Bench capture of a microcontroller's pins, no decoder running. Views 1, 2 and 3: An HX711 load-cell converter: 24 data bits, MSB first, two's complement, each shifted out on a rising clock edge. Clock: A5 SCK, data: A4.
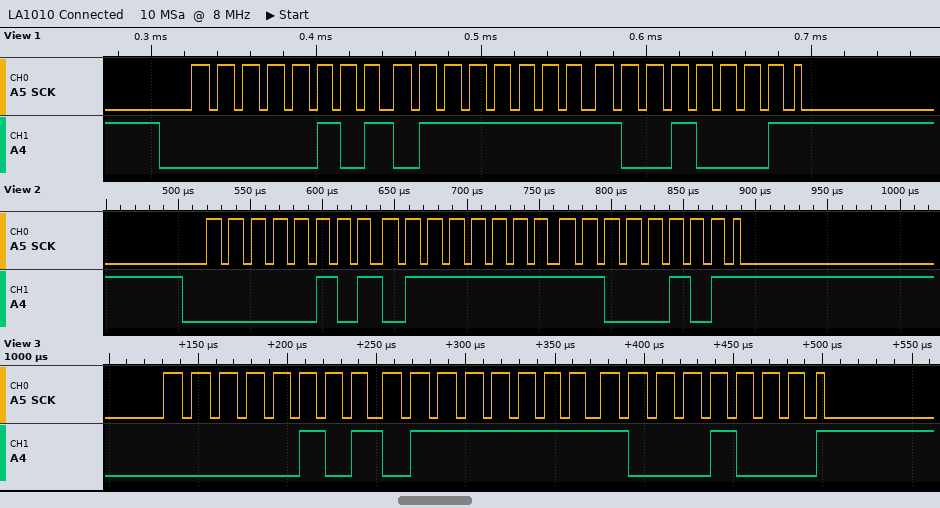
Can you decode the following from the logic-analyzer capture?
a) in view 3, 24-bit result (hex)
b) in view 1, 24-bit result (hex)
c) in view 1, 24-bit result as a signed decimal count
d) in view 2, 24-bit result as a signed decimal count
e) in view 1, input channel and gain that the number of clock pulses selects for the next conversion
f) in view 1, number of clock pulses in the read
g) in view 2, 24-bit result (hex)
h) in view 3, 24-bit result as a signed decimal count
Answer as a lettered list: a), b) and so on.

a) 0x057F88
b) 0x057F91
c) 360337
d) 360389
e) channel A, gain 128
f) 25
g) 0x057FC5
h) 360328
